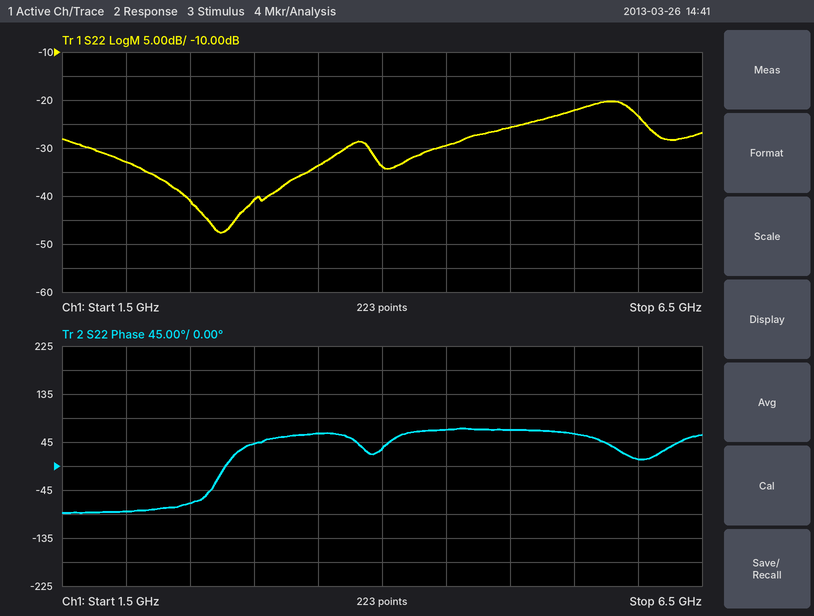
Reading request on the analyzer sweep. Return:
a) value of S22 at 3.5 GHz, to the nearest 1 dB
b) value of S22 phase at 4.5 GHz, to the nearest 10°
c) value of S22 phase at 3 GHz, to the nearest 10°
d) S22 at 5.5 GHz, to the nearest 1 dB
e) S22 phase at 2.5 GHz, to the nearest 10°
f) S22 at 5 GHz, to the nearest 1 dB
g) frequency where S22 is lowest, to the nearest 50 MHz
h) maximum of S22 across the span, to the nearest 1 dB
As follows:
-34 dB
70°
40°
-22 dB
-70°
-26 dB
2.75 GHz
-20 dB
